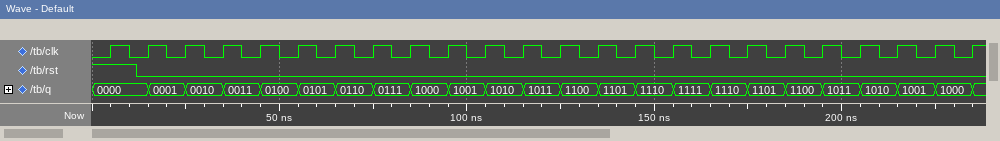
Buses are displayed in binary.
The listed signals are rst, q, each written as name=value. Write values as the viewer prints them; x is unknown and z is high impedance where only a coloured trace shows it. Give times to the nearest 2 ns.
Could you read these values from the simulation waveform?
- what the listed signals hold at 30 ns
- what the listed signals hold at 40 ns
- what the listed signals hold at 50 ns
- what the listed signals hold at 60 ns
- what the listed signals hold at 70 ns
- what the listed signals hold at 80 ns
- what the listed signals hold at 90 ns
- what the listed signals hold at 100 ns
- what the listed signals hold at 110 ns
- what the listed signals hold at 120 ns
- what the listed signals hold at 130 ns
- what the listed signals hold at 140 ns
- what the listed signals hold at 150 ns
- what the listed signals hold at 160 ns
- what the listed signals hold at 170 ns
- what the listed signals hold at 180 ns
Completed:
rst=0, q=0010
rst=0, q=0011
rst=0, q=0100
rst=0, q=0101
rst=0, q=0110
rst=0, q=0111
rst=0, q=1000
rst=0, q=1001
rst=0, q=1010
rst=0, q=1011
rst=0, q=1100
rst=0, q=1101
rst=0, q=1110
rst=0, q=1111
rst=0, q=1110
rst=0, q=1101
